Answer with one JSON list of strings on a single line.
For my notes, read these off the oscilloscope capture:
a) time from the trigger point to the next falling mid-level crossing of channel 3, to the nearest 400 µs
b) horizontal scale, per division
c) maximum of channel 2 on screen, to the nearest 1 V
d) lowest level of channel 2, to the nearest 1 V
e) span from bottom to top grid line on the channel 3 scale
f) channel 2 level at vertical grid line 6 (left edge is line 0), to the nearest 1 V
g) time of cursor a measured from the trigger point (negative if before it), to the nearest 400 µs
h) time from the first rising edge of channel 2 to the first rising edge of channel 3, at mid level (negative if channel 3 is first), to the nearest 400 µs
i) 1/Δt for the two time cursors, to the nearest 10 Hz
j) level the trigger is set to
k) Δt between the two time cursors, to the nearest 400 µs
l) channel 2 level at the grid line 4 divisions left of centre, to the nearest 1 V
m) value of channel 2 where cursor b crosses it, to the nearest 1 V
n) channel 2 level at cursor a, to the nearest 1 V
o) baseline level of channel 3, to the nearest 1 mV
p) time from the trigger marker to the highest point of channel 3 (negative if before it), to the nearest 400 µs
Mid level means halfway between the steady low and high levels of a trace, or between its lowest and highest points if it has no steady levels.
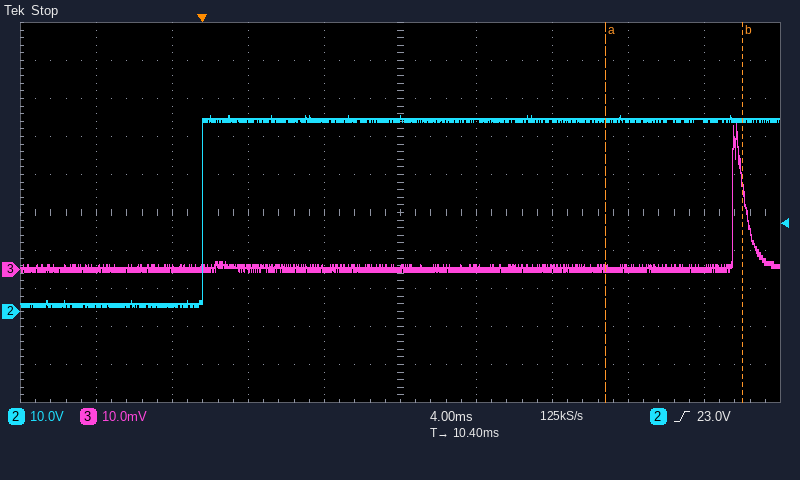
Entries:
["28.4 ms", "4 ms", "52 V", "1 V", "100 mV", "50 V", "+21.2 ms", "+28.0 ms", "140 Hz", "23.0 V", "7.2 ms", "2 V", "50 V", "50 V", "0 mV", "+28.0 ms"]
